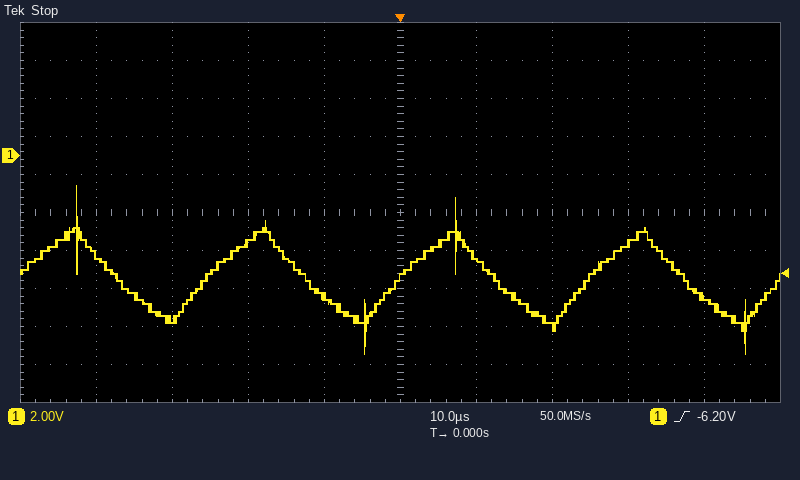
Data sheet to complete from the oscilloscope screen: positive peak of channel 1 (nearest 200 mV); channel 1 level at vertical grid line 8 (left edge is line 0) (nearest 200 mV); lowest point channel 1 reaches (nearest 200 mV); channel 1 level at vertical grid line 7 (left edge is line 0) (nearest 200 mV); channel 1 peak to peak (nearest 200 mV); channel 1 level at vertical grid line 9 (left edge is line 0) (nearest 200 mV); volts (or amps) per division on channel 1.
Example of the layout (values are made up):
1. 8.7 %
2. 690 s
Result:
1. -1.6 V
2. -4.6 V
3. -10.4 V
4. -9.0 V
5. 8.8 V
6. -7.4 V
7. 2 V
